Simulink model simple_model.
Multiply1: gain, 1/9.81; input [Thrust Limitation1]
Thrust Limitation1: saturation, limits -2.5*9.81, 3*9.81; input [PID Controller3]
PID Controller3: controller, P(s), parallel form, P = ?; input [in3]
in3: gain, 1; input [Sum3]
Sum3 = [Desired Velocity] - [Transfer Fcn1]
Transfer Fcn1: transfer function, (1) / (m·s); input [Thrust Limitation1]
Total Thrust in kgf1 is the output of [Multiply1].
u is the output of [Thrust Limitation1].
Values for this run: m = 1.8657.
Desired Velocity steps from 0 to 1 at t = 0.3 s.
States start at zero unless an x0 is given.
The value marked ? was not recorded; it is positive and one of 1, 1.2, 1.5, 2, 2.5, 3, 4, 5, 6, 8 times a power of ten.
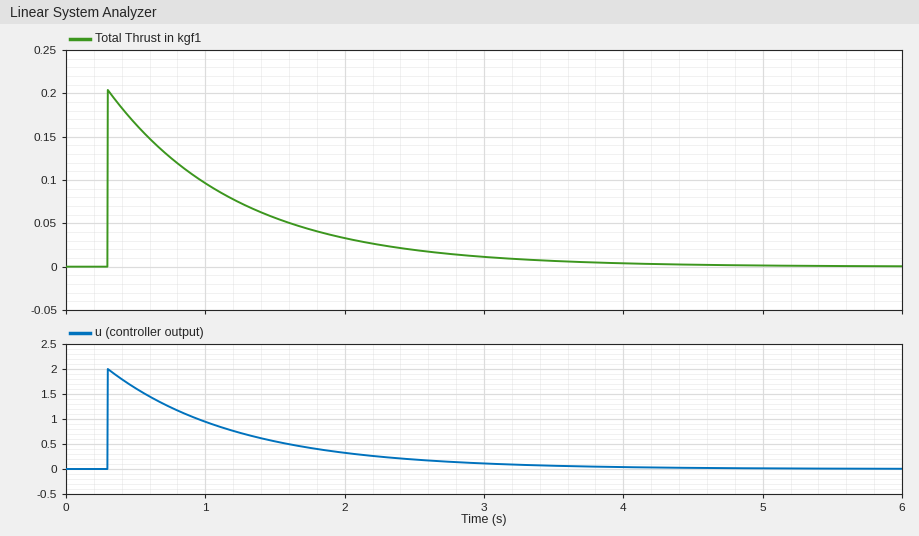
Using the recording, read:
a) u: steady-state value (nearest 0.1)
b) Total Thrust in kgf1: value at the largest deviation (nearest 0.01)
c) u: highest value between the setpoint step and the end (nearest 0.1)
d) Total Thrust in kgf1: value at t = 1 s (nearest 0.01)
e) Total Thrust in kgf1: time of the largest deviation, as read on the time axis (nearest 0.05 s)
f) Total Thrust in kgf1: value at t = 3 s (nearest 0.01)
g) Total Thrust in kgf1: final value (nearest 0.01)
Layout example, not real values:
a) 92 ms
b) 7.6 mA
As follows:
a) 0.0
b) 0.20
c) 2.0
d) 0.10
e) 0.30 s
f) 0.01
g) 0.00
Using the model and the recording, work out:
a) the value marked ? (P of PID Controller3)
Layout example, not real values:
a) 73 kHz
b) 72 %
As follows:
a) 2
